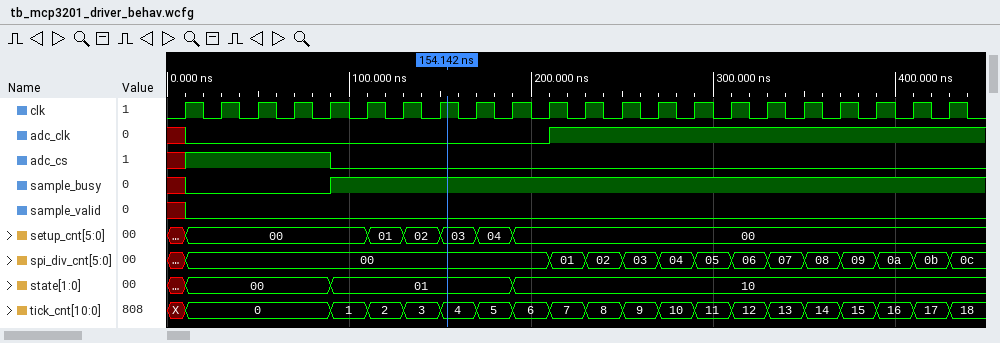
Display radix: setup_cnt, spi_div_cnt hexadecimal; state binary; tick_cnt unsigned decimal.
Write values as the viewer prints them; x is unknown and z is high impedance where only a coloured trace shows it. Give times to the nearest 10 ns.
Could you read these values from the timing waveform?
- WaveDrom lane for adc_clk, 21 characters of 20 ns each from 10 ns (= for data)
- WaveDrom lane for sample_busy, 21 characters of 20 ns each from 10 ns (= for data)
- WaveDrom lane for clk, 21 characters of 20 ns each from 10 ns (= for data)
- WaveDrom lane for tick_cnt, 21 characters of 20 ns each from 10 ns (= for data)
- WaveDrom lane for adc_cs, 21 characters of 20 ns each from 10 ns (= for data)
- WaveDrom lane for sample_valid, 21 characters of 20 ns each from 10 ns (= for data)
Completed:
{name: 'adc_clk', wave: '0.........1..........'}
{name: 'sample_busy', wave: '0...1................'}
{name: 'clk', wave: 'p....................'}
{name: 'tick_cnt', wave: '=...=================', data: '0 1 2 3 4 5 6 7 8 9 10 11 12 13 14 15 16 17'}
{name: 'adc_cs', wave: '1...0................'}
{name: 'sample_valid', wave: '0....................'}
